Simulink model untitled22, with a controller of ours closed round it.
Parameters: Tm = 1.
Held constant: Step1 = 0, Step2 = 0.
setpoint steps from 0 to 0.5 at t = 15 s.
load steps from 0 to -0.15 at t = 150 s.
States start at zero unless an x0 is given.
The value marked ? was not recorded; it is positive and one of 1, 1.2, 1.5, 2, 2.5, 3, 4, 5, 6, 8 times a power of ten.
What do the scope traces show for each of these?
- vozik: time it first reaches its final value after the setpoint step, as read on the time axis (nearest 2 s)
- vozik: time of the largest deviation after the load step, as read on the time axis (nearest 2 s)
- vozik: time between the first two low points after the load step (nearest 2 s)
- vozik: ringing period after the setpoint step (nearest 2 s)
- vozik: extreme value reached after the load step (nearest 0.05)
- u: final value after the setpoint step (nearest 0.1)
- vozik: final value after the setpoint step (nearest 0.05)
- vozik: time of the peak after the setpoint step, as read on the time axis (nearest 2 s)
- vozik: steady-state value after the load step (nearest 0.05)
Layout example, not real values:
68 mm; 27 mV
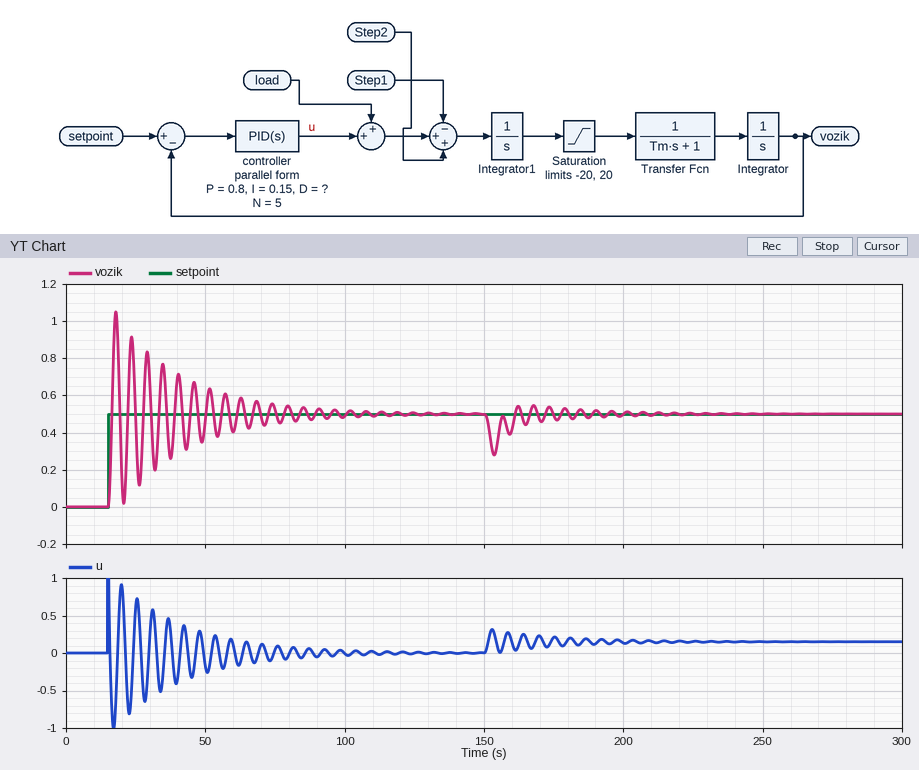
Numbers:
16 s; 154 s; 6 s; 6 s; 0.30; 0.0; 0.50; 18 s; 0.50
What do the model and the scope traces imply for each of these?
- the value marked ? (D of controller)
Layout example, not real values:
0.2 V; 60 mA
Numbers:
1.5
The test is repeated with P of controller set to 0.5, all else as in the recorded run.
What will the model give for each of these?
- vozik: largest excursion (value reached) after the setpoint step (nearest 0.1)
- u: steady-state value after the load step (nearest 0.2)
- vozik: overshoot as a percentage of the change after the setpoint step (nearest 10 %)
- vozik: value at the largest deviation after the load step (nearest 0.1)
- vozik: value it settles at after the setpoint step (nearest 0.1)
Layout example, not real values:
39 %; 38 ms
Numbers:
1.0; 0.2; 90 %; 0.2; 0.5
